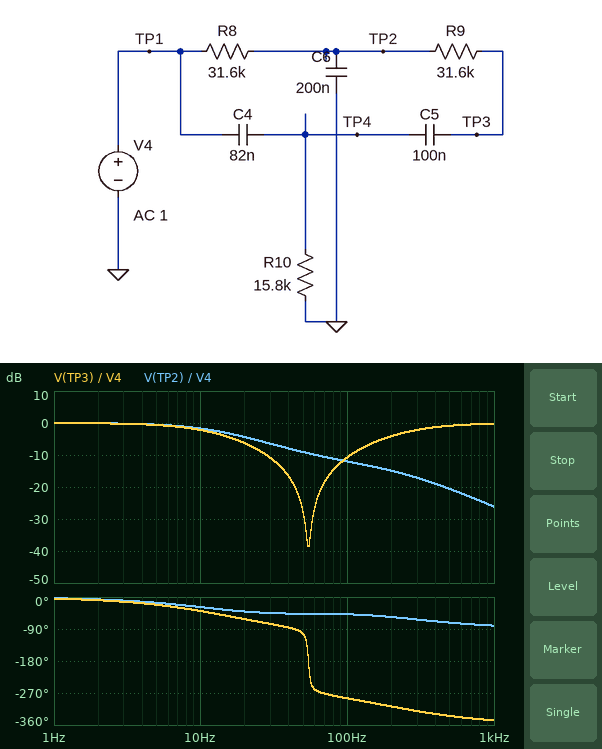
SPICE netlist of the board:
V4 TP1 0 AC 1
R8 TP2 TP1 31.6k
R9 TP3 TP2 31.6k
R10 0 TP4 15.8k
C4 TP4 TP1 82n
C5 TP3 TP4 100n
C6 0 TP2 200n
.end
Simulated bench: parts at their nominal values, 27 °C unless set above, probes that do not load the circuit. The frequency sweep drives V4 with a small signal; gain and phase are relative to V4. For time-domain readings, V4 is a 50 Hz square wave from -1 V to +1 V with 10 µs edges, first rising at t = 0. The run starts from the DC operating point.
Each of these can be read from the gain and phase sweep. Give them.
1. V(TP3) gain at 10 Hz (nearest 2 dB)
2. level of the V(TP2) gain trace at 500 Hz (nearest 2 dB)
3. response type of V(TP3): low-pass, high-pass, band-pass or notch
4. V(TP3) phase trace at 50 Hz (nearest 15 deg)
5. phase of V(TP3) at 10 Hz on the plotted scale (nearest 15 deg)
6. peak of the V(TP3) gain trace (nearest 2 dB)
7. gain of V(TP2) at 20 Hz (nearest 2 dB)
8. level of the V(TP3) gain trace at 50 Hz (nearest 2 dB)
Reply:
-2 dB
-20 dB
notch
-105 deg
-45 deg
0 dB
-4 dB
-28 dB
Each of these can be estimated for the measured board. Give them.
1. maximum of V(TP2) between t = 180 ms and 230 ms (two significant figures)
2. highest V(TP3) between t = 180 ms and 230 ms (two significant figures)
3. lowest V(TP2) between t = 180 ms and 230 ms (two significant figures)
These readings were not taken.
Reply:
530 mV
1.7 V
-530 mV
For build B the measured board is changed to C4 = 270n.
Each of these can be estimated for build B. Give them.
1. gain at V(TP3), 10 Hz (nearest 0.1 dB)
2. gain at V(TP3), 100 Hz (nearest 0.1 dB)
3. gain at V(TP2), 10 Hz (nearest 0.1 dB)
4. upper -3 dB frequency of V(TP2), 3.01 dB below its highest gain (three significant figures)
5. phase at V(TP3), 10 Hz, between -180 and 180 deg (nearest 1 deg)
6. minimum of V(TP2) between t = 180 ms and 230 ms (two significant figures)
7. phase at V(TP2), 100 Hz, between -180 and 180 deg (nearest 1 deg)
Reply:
-2.8 dB
-4.5 dB
-1.9 dB
13.6 Hz
-38 deg
-550 mV
-47 deg
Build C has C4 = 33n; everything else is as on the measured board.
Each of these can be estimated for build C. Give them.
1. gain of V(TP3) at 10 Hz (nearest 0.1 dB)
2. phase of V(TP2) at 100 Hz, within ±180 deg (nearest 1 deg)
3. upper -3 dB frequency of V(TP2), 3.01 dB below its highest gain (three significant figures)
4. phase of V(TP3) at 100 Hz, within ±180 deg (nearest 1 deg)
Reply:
-2.0 dB
-58 deg
15.1 Hz
103 deg
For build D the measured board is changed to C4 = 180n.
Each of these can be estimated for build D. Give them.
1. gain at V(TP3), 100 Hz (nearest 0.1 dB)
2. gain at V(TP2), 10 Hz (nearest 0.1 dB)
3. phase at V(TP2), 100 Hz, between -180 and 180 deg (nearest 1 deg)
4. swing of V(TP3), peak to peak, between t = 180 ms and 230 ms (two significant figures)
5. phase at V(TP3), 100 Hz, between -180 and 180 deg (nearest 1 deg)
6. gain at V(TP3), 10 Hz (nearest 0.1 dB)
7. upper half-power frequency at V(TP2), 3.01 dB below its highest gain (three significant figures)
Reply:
-5.9 dB
-1.8 dB
-46 deg
3.4 V
54 deg
-2.5 dB
14.0 Hz
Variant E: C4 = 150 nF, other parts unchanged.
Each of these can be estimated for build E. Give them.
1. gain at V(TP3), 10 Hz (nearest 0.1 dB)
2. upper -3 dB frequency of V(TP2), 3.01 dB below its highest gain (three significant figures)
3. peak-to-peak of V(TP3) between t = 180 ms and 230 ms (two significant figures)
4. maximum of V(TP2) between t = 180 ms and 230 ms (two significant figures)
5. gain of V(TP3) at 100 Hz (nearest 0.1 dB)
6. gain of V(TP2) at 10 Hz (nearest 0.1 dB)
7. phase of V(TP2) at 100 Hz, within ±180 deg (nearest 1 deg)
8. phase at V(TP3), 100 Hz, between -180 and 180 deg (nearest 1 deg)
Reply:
-2.4 dB
14.1 Hz
3.4 V
530 mV
-6.7 dB
-1.8 dB
-46 deg
59 deg
